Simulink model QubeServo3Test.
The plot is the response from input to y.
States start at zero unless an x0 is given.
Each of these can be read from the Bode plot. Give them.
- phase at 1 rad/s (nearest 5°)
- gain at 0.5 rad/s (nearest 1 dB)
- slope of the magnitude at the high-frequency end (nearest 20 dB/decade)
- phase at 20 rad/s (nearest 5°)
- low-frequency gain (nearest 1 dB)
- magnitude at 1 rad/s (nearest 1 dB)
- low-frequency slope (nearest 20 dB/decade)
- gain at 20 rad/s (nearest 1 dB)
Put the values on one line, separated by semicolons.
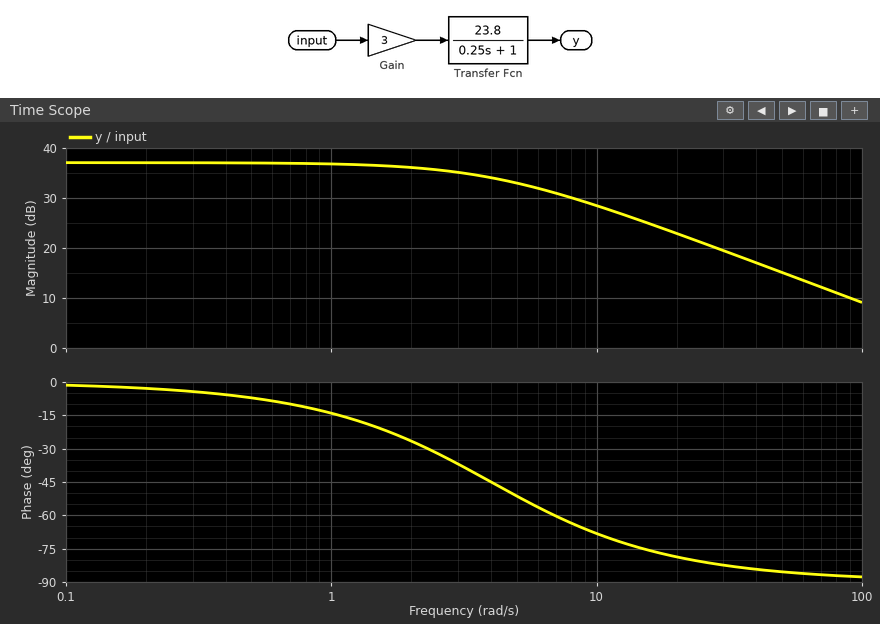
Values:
-15°; 37 dB; -20 dB/decade; -80°; 37 dB; 37 dB; 0 dB/decade; 23 dB
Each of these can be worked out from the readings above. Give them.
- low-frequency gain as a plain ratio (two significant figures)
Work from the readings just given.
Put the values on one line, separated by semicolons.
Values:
71
